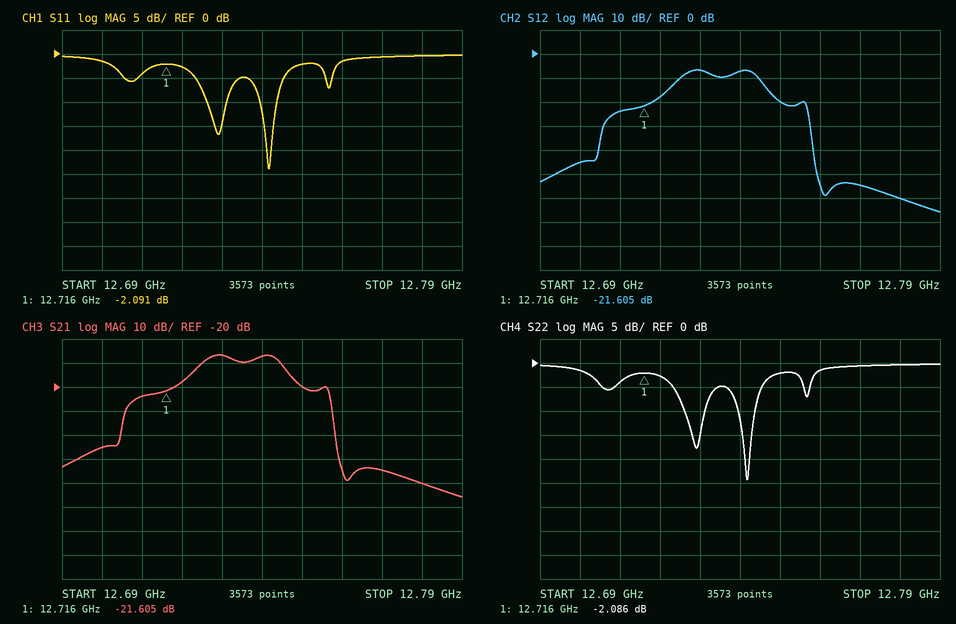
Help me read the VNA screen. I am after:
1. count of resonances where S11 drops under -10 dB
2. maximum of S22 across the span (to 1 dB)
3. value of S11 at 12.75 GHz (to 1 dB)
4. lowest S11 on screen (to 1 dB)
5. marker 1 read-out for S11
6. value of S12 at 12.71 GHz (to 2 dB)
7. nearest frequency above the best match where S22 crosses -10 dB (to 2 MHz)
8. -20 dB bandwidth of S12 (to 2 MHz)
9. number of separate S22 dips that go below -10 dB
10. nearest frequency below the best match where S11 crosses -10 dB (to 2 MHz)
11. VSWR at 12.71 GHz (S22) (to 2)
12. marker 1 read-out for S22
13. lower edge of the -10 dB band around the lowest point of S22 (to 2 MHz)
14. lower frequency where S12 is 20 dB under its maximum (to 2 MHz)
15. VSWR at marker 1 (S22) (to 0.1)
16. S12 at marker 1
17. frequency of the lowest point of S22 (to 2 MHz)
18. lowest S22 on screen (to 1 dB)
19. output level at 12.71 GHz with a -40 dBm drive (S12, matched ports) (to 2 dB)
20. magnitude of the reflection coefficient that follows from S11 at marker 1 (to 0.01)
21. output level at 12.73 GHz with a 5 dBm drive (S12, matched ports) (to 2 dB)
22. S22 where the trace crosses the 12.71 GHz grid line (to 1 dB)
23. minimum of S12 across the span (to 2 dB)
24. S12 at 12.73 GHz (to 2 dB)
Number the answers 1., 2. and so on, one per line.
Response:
1. 2
2. 0 dB
3. -2 dB
4. -24 dB
5. -2.091 dB
6. -24 dB
7. 12.744 GHz
8. 50 MHz
9. 2
10. 12.740 GHz
11. 4
12. -2.086 dB
13. 12.740 GHz
14. 12.708 GHz
15. 8.4
16. -21.605 dB
17. 12.742 GHz
18. -24 dB
19. -64 dBm
20. 0.79
21. -2 dBm
22. -4 dB
23. -66 dB
24. -6 dB
